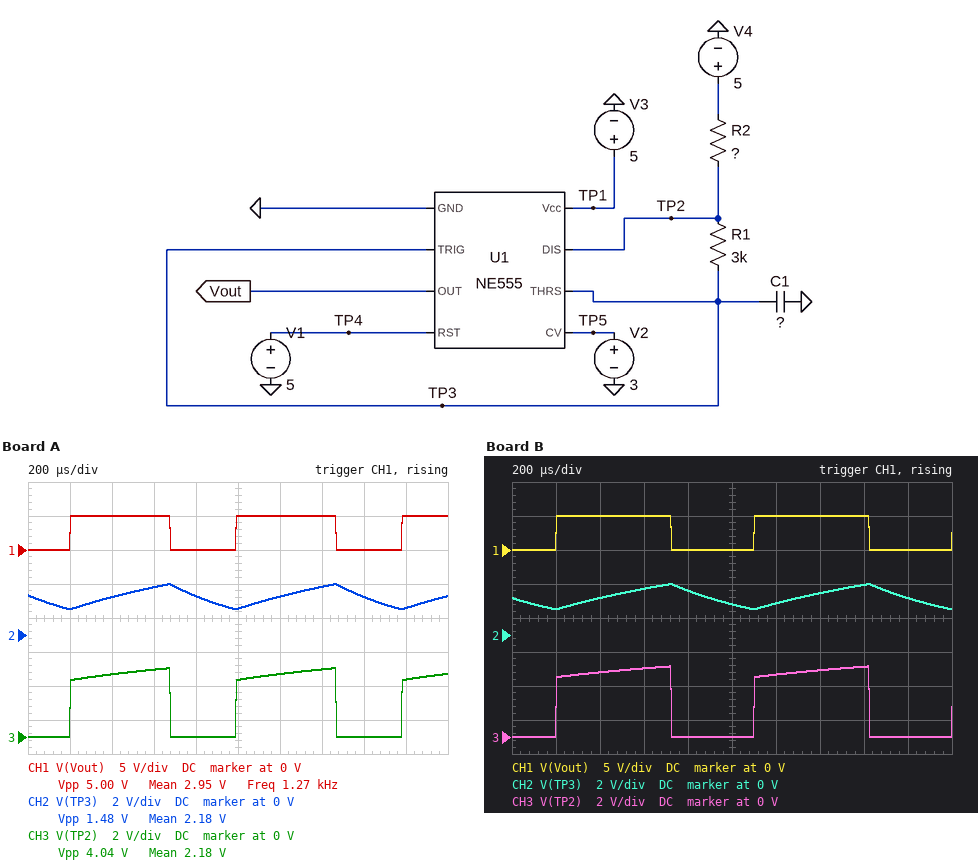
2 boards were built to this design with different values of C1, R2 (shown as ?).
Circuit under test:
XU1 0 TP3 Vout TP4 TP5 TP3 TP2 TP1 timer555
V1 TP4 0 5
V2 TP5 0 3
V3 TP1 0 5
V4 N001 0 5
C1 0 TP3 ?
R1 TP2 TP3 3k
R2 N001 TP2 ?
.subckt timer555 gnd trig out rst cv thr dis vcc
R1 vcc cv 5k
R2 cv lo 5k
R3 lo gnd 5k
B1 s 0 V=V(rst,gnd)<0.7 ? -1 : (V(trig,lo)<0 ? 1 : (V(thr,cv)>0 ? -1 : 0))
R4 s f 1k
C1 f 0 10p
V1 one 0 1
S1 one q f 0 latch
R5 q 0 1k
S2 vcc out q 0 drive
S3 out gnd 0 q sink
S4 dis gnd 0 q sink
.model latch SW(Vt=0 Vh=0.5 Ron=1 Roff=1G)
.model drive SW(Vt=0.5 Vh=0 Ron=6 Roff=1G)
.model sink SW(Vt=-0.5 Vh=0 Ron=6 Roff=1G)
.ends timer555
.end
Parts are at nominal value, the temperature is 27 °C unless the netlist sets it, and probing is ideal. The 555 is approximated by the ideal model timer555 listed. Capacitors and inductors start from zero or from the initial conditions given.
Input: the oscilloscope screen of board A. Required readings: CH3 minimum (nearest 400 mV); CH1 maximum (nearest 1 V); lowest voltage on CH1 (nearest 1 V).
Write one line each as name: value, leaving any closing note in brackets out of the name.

CH3 minimum: 0 V
CH1 maximum: 5 V
lowest voltage on CH1: 0 V
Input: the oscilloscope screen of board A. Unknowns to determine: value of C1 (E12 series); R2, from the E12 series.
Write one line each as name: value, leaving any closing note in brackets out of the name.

value of C1: 150 nF
R2, from the E12 series: 2.7 kΩ
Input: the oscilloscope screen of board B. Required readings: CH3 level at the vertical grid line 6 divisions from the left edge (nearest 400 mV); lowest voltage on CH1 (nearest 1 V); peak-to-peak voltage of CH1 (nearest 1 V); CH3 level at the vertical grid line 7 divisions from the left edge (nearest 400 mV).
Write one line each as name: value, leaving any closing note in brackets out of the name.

CH3 level at the vertical grid line 6 divisions from the left edge: 3.6 V
lowest voltage on CH1: 0 V
peak-to-peak voltage of CH1: 5 V
CH3 level at the vertical grid line 7 divisions from the left edge: 4.0 V
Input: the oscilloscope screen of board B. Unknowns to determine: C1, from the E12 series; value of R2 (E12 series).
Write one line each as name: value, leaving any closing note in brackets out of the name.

C1, from the E12 series: 180 nF
value of R2: 2.2 kΩ
